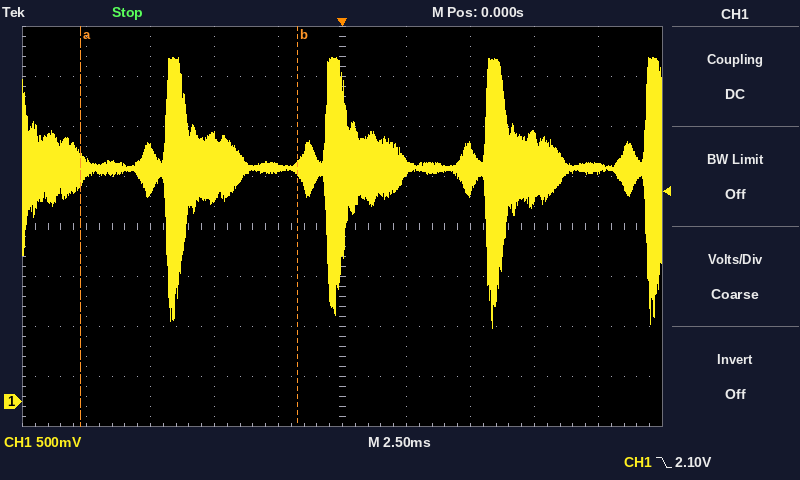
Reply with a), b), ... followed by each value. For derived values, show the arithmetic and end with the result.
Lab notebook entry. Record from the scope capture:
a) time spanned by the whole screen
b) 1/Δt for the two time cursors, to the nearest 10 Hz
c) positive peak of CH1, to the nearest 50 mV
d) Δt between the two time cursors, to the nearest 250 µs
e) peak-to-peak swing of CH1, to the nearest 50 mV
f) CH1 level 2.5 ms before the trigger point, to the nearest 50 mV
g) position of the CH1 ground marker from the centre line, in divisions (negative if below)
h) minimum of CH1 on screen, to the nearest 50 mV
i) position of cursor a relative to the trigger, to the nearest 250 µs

a) 25 ms
b) 1 / 8.50 ms ≈ 120 Hz
c) 3.45 V
d) 8.50 ms
e) 3.45 V − (750 mV) = 2.70 V
f) 2.35 V
g) -3.5 div
h) 750 mV
i) -10.25 ms
